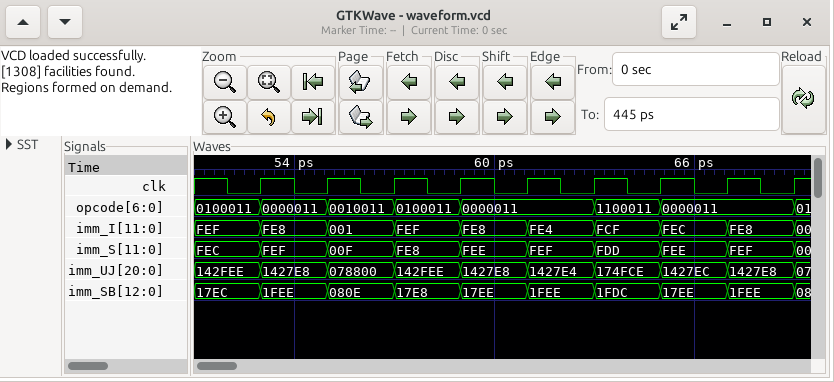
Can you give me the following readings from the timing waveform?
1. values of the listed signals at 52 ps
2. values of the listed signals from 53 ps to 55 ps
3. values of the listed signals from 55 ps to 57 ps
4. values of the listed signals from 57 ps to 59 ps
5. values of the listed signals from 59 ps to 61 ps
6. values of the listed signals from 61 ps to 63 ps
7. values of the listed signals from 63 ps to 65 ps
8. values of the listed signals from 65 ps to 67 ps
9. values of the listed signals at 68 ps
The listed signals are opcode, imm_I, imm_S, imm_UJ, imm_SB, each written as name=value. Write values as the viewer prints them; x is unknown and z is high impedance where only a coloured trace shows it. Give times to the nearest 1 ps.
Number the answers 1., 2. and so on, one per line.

1. opcode=0100011, imm_I=FEF, imm_S=FEC, imm_UJ=142FEE, imm_SB=17EC
2. opcode=0000011, imm_I=FE8, imm_S=FEF, imm_UJ=1427E8, imm_SB=1FEE
3. opcode=0010011, imm_I=001, imm_S=00F, imm_UJ=078800, imm_SB=080E
4. opcode=0100011, imm_I=FEF, imm_S=FE8, imm_UJ=142FEE, imm_SB=17E8
5. opcode=0000011, imm_I=FE8, imm_S=FEE, imm_UJ=1427E8, imm_SB=17EE
6. opcode=0000011, imm_I=FE4, imm_S=FEF, imm_UJ=1427E4, imm_SB=1FEE
7. opcode=1100011, imm_I=FCF, imm_S=FDD, imm_UJ=174FCE, imm_SB=1FDC
8. opcode=0000011, imm_I=FEC, imm_S=FEE, imm_UJ=1427EC, imm_SB=17EE
9. opcode=0000011, imm_I=FE8, imm_S=FEF, imm_UJ=1427E8, imm_SB=1FEE
